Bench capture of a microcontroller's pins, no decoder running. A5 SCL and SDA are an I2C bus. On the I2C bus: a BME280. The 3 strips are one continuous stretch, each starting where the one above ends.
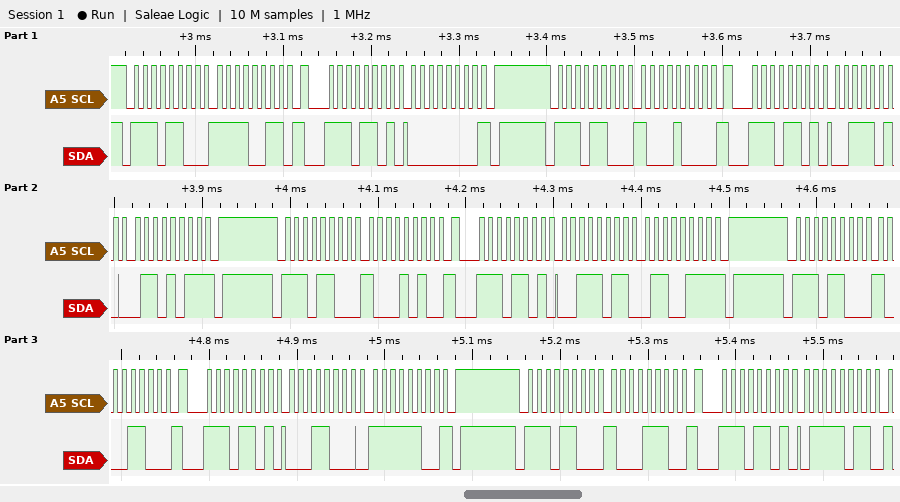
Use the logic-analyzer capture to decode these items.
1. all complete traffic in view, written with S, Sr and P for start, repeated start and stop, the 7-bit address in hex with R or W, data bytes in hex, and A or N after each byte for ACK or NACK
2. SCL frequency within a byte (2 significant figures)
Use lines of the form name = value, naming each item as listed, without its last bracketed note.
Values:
all complete traffic in view, written with S, Sr and P for start, repeated start and stop, the 7-bit address in hex with R or W, data bytes in hex, and A or N after each byte for ACK or NACK = S 76W A F3 A Sr 76R A 00 N P S 76W A 88 A Sr 76R A 3A A 6B N P S 76W A 8A A Sr 76R A 3B A 67 N P S 76W A 8C A Sr 76R A 18 A FC N P S 76W A 8E A Sr 76R A 7B A
SCL frequency within a byte = 100 kHz
